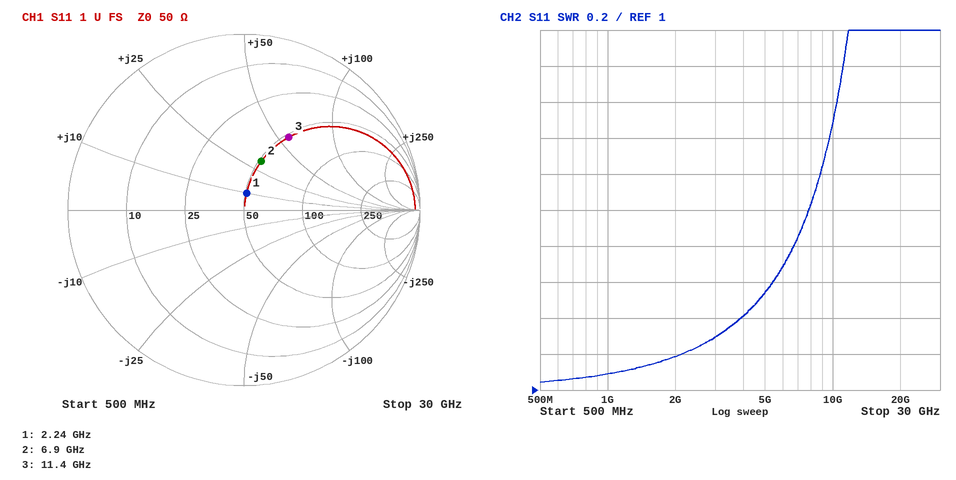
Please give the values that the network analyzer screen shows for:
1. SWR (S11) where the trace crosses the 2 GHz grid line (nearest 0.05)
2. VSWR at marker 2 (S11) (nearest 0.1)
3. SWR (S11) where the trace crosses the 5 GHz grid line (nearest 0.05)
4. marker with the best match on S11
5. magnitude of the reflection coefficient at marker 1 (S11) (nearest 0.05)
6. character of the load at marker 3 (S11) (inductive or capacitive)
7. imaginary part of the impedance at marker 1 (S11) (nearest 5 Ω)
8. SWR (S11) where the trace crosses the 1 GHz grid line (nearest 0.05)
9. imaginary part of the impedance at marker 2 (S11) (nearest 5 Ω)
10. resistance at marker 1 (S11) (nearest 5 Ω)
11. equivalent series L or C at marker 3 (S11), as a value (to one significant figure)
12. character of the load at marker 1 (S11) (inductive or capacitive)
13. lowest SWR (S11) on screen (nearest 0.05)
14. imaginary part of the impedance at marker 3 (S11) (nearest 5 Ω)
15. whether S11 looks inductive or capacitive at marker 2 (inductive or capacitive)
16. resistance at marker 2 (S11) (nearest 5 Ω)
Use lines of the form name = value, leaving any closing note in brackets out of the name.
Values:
SWR (S11) where the trace crosses the 2 GHz grid line = 1.20
VSWR at marker 2 (S11) = 1.8
SWR (S11) where the trace crosses the 5 GHz grid line = 1.55
marker with the best match on S11 = marker 1
magnitude of the reflection coefficient at marker 1 (S11) = 0.10
character of the load at marker 3 (S11) = inductive
imaginary part of the impedance at marker 1 (S11) = +10 Ω
SWR (S11) where the trace crosses the 1 GHz grid line = 1.10
imaginary part of the impedance at marker 2 (S11) = +30 Ω
resistance at marker 1 (S11) = 50 Ω
equivalent series L or C at marker 3 (S11), as a value = 800 pH
character of the load at marker 1 (S11) = inductive
lowest SWR (S11) on screen = 1.05
imaginary part of the impedance at marker 3 (S11) = +55 Ω
whether S11 looks inductive or capacitive at marker 2 = inductive
resistance at marker 2 (S11) = 50 Ω
